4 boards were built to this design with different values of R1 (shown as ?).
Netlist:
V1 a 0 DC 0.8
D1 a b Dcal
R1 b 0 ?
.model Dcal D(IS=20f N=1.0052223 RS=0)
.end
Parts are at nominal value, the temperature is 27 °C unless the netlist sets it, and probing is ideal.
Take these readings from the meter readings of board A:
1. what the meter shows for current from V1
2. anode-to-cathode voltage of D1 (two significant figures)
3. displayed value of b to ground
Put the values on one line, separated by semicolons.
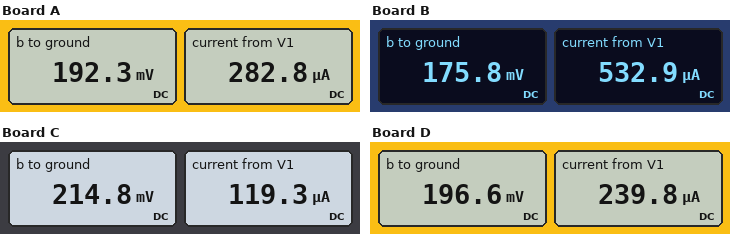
282.8 µA; 610 mV; 192.3 mV
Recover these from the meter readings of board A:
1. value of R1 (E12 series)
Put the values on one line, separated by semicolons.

680 Ω
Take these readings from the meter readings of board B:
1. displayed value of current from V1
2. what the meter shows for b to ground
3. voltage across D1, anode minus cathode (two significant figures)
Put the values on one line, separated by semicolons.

532.9 µA; 175.8 mV; 620 mV
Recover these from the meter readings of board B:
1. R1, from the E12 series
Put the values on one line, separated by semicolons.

330 Ω
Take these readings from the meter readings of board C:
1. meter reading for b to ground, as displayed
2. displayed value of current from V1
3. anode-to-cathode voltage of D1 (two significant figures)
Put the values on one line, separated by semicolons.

214.8 mV; 119.3 µA; 590 mV
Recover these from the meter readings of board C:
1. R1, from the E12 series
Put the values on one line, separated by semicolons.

1.8 kΩ
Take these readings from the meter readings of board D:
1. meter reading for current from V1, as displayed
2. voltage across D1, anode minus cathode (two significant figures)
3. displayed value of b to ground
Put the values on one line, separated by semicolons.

239.8 µA; 600 mV; 196.6 mV
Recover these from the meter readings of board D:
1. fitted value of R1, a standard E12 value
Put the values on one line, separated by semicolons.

820 Ω
